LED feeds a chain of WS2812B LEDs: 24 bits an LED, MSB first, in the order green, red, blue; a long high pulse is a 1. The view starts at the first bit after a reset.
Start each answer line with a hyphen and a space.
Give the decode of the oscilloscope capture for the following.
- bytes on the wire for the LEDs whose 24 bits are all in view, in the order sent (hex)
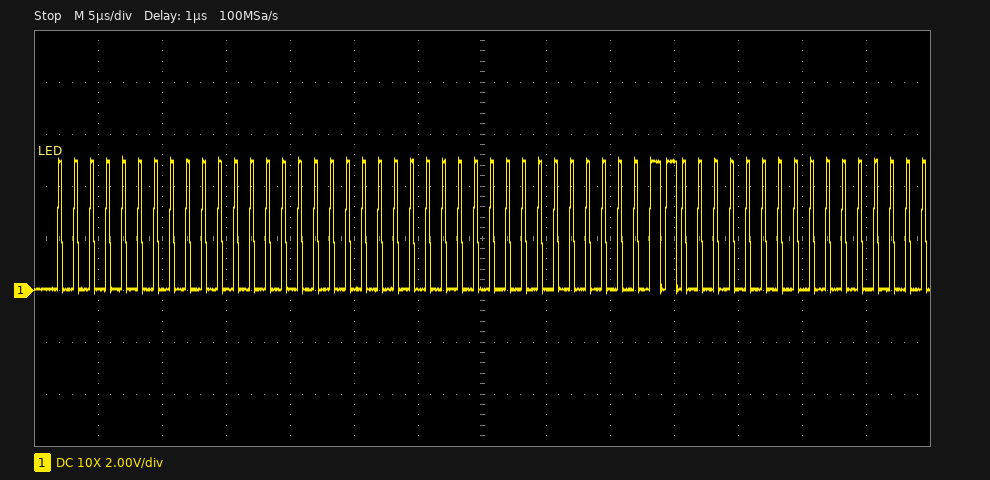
- 00 00 00 00 06 00
